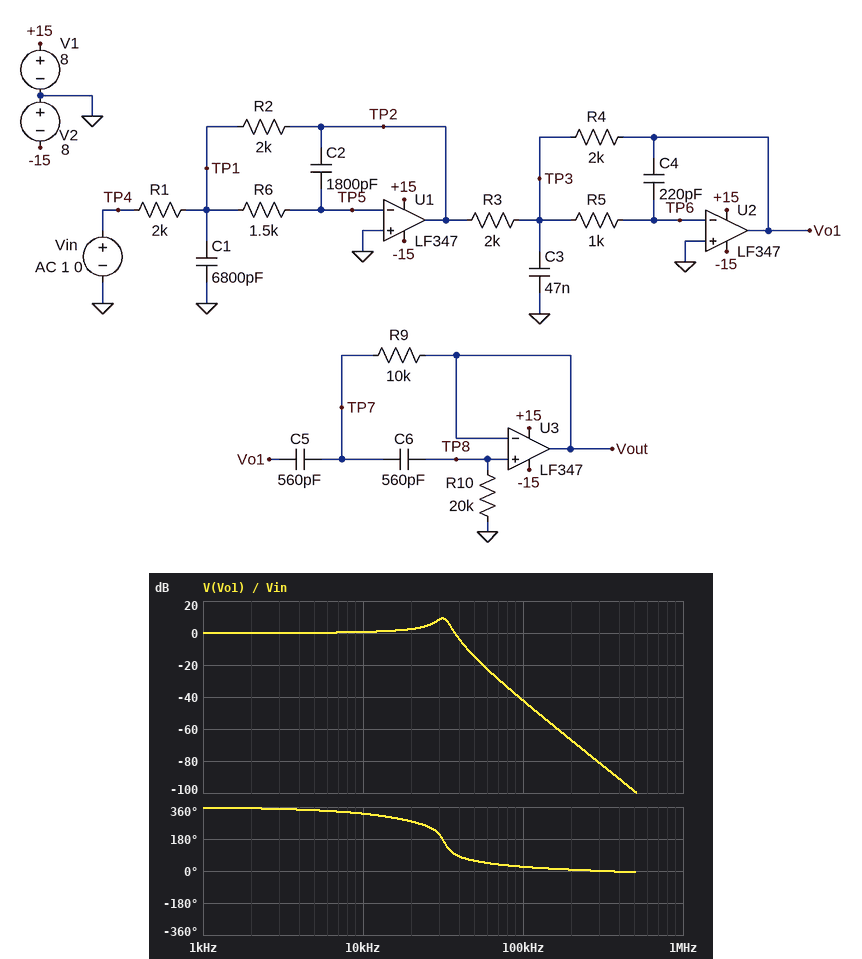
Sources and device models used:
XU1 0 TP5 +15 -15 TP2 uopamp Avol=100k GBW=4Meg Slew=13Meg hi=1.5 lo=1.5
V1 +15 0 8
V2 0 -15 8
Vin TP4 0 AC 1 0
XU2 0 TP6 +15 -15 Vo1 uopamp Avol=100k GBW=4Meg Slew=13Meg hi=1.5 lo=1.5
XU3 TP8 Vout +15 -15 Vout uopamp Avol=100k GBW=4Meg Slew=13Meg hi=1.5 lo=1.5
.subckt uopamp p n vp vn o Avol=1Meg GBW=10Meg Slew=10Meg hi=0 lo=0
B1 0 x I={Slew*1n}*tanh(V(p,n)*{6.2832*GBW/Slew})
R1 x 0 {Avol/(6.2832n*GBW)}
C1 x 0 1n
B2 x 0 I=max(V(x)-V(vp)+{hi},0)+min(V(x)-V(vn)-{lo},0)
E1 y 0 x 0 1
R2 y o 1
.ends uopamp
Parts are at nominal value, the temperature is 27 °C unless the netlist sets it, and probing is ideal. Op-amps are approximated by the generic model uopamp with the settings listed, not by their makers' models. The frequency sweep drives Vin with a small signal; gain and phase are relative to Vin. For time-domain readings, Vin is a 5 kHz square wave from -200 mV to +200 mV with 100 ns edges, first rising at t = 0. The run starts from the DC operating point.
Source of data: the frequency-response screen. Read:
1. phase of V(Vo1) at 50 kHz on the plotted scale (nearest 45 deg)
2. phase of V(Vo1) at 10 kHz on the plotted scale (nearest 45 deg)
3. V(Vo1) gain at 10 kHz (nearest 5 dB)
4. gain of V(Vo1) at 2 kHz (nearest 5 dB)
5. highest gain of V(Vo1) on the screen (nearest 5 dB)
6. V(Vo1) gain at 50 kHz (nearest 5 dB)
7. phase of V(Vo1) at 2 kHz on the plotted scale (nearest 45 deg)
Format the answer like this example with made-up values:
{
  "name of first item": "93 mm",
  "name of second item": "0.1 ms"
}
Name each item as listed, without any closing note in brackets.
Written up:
{
  "phase of V(Vo1) at 50 kHz on the plotted scale": "45 deg",
  "phase of V(Vo1) at 10 kHz on the plotted scale": "315 deg",
  "V(Vo1) gain at 10 kHz": "0 dB",
  "gain of V(Vo1) at 2 kHz": "0 dB",
  "highest gain of V(Vo1) on the screen": "10 dB",
  "V(Vo1) gain at 50 kHz": "-15 dB",
  "phase of V(Vo1) at 2 kHz on the plotted scale": "360 deg"
}
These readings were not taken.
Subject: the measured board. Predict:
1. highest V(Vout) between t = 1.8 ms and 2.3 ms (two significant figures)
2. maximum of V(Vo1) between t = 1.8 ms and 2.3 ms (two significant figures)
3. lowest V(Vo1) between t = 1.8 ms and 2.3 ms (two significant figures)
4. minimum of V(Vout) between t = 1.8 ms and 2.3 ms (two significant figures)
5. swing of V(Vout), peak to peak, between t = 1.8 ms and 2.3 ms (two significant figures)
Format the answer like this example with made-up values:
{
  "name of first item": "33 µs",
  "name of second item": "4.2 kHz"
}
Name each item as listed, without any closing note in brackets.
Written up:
{
  "highest V(Vout) between t = 1.8 ms and 2.3 ms": "180 mV",
  "maximum of V(Vo1) between t = 1.8 ms and 2.3 ms": "360 mV",
  "lowest V(Vo1) between t = 1.8 ms and 2.3 ms": "-360 mV",
  "minimum of V(Vout) between t = 1.8 ms and 2.3 ms": "-180 mV",
  "swing of V(Vout), peak to peak, between t = 1.8 ms and 2.3 ms": "360 mV"
}
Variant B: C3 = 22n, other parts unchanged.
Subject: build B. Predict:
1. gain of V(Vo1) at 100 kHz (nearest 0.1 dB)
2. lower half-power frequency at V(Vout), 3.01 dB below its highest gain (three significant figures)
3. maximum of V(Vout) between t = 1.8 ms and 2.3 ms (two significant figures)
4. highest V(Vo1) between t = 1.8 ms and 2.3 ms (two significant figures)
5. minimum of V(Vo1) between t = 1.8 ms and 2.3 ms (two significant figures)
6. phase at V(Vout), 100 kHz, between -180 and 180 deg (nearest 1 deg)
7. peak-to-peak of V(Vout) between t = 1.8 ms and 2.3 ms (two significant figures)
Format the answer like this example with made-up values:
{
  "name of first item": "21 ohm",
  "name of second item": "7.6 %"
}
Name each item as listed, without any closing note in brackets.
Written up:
{
  "gain of V(Vo1) at 100 kHz": "-34.5 dB",
  "lower half-power frequency at V(Vout), 3.01 dB below its highest gain": "23.1 kHz",
  "maximum of V(Vout) between t = 1.8 ms and 2.3 ms": "150 mV",
  "highest V(Vo1) between t = 1.8 ms and 2.3 ms": "260 mV",
  "minimum of V(Vo1) between t = 1.8 ms and 2.3 ms": "-260 mV",
  "phase at V(Vout), 100 kHz, between -180 and 180 deg": "44 deg",
  "peak-to-peak of V(Vout) between t = 1.8 ms and 2.3 ms": "290 mV"
}
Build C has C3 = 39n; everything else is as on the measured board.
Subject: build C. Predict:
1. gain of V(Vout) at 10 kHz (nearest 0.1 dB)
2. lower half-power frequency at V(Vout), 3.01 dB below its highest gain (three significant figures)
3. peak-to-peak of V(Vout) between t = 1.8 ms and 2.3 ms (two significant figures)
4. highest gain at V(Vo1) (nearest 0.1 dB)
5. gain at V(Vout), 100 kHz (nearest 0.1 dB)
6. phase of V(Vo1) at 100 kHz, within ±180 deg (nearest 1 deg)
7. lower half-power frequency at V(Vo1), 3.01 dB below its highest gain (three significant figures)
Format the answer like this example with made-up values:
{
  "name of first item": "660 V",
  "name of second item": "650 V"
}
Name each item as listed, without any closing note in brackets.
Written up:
{
  "gain of V(Vout) at 10 kHz": "-11.9 dB",
  "lower half-power frequency at V(Vout), 3.01 dB below its highest gain": "29.6 kHz",
  "peak-to-peak of V(Vout) between t = 1.8 ms and 2.3 ms": "380 mV",
  "highest gain at V(Vo1)": "7.3 dB",
  "gain at V(Vout), 100 kHz": "-40.4 dB",
  "phase of V(Vo1) at 100 kHz, within ±180 deg": "25 deg",
  "lower half-power frequency at V(Vo1), 3.01 dB below its highest gain": "29.0 kHz"
}
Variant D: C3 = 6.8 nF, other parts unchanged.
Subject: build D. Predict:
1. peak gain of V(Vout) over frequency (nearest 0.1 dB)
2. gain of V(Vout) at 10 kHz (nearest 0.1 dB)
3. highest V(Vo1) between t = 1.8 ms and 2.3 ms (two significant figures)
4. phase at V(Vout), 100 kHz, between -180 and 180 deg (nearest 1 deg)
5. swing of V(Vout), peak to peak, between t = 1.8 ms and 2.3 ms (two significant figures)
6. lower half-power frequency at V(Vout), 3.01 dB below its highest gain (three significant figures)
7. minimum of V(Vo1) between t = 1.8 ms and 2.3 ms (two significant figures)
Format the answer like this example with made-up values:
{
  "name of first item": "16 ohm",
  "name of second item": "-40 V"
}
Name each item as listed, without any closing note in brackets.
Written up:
{
  "peak gain of V(Vout) over frequency": "-3.9 dB",
  "gain of V(Vout) at 10 kHz": "-12.5 dB",
  "highest V(Vo1) between t = 1.8 ms and 2.3 ms": "210 mV",
  "phase at V(Vout), 100 kHz, between -180 and 180 deg": "91 deg",
  "swing of V(Vout), peak to peak, between t = 1.8 ms and 2.3 ms": "240 mV",
  "lower half-power frequency at V(Vout), 3.01 dB below its highest gain": "14.8 kHz",
  "minimum of V(Vo1) between t = 1.8 ms and 2.3 ms": "-210 mV"
}
